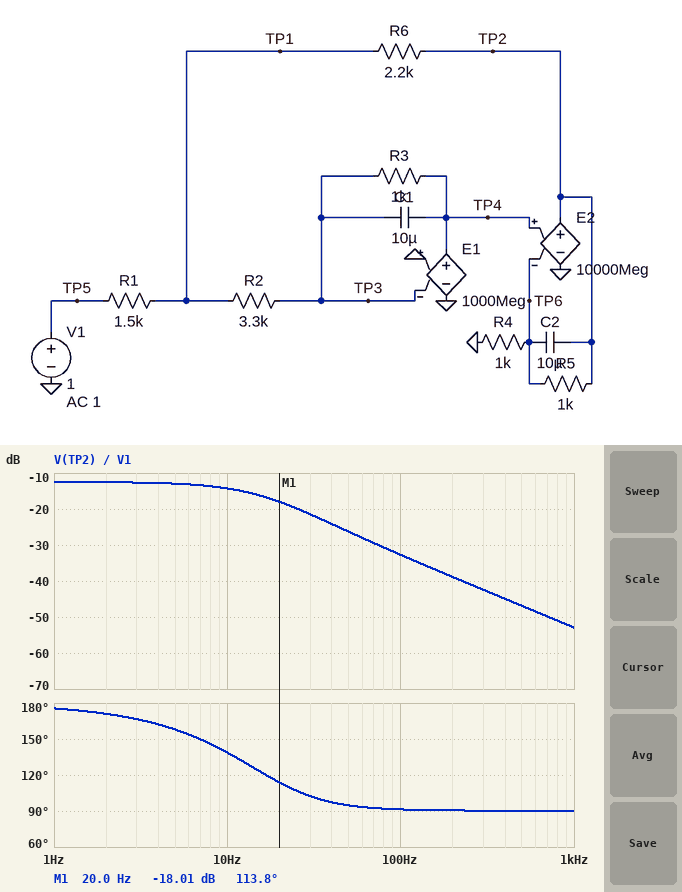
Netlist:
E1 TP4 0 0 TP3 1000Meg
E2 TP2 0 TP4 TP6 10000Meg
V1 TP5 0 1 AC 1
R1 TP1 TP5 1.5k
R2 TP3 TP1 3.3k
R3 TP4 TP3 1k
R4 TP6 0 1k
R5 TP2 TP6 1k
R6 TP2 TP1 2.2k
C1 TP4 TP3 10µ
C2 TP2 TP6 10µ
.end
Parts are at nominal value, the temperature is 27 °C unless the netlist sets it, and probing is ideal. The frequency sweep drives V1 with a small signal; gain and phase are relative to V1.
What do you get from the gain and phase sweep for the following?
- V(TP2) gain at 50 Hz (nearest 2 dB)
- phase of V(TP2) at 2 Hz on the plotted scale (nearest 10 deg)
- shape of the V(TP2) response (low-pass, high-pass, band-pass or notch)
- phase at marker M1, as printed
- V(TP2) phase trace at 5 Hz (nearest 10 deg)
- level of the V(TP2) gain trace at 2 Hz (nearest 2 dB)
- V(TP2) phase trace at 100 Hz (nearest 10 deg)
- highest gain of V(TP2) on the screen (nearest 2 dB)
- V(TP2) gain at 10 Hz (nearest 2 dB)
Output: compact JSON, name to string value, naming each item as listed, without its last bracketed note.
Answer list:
{"V(TP2) gain at 50 Hz": "-26 dB", "phase of V(TP2) at 2 Hz on the plotted scale": "170 deg", "shape of the V(TP2) response": "low-pass", "phase at marker M1, as printed": "113.8 deg", "V(TP2) phase trace at 5 Hz": "160 deg", "level of the V(TP2) gain trace at 2 Hz": "-12 dB", "V(TP2) phase trace at 100 Hz": "90 deg", "highest gain of V(TP2) on the screen": "-12 dB", "V(TP2) gain at 10 Hz": "-14 dB"}
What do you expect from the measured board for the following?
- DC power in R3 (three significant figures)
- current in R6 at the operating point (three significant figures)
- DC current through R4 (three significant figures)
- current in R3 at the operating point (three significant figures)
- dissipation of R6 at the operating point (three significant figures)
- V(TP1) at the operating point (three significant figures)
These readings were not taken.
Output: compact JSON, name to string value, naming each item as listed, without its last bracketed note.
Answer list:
{"DC power in R3": "14.1 µW", "current in R6 at the operating point": "286 µA", "DC current through R4": "119 µA", "current in R3 at the operating point": "119 µA", "dissipation of R6 at the operating point": "180 µW", "V(TP1) at the operating point": "392 mV"}
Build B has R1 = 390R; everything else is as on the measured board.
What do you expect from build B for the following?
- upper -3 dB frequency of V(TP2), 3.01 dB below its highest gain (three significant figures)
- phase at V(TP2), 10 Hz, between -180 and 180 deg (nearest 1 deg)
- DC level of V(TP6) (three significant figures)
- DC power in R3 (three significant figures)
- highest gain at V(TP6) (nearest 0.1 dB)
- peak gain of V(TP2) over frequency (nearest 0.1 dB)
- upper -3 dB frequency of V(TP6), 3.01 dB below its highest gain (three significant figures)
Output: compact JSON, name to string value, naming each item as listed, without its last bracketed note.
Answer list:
{"upper -3 dB frequency of V(TP2), 3.01 dB below its highest gain": "12.2 Hz", "phase at V(TP2), 10 Hz, between -180 and 180 deg": "136 deg", "DC level of V(TP6)": "-216 mV", "DC power in R3": "46.7 µW", "highest gain at V(TP6)": "-13.3 dB", "peak gain of V(TP2) over frequency": "-7.3 dB", "upper -3 dB frequency of V(TP6), 3.01 dB below its highest gain": "17.9 Hz"}
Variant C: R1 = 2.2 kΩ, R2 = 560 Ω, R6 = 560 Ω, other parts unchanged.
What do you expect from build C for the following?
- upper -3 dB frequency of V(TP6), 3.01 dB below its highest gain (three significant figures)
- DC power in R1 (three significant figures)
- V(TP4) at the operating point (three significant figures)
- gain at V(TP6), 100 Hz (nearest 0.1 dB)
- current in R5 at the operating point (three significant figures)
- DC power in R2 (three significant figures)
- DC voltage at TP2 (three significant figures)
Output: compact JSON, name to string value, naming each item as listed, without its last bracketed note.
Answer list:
{"upper -3 dB frequency of V(TP6), 3.01 dB below its highest gain": "45.2 Hz", "DC power in R1": "416 µW", "V(TP4) at the operating point": "-78.0 mV", "gain at V(TP6), 100 Hz": "-30.1 dB", "current in R5 at the operating point": "78.0 µA", "DC power in R2": "3.41 µW", "DC voltage at TP2": "-156 mV"}
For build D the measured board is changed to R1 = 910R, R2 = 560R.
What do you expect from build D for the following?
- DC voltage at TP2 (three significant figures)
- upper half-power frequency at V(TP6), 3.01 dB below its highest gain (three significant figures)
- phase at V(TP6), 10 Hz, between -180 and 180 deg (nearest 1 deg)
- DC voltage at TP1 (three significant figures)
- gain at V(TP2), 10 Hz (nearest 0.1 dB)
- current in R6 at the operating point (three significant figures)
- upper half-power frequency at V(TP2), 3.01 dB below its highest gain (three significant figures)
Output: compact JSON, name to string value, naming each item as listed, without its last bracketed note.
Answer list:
{"DC voltage at TP2": "-791 mV", "upper half-power frequency at V(TP6), 3.01 dB below its highest gain": "27.9 Hz", "phase at V(TP6), 10 Hz, between -180 and 180 deg": "160 deg", "DC voltage at TP1": "221 mV", "gain at V(TP2), 10 Hz": "-3.2 dB", "current in R6 at the operating point": "460 µA", "upper half-power frequency at V(TP2), 3.01 dB below its highest gain": "16.6 Hz"}
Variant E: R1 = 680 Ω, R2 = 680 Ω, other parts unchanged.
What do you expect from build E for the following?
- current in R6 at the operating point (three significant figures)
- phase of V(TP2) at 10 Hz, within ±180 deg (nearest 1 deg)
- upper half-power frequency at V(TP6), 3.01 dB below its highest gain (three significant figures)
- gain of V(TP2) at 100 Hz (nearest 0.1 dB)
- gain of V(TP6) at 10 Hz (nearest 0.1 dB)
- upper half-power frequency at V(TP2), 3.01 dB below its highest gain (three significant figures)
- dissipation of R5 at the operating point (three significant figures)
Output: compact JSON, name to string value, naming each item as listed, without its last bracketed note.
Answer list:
{"current in R6 at the operating point": "557 µA", "phase of V(TP2) at 10 Hz, within ±180 deg": "143 deg", "upper half-power frequency at V(TP6), 3.01 dB below its highest gain": "25.6 Hz", "gain of V(TP2) at 100 Hz": "-19.7 dB", "gain of V(TP6) at 10 Hz": "-7.1 dB", "upper half-power frequency at V(TP2), 3.01 dB below its highest gain": "15.6 Hz", "dissipation of R5 at the operating point": "209 µW"}
